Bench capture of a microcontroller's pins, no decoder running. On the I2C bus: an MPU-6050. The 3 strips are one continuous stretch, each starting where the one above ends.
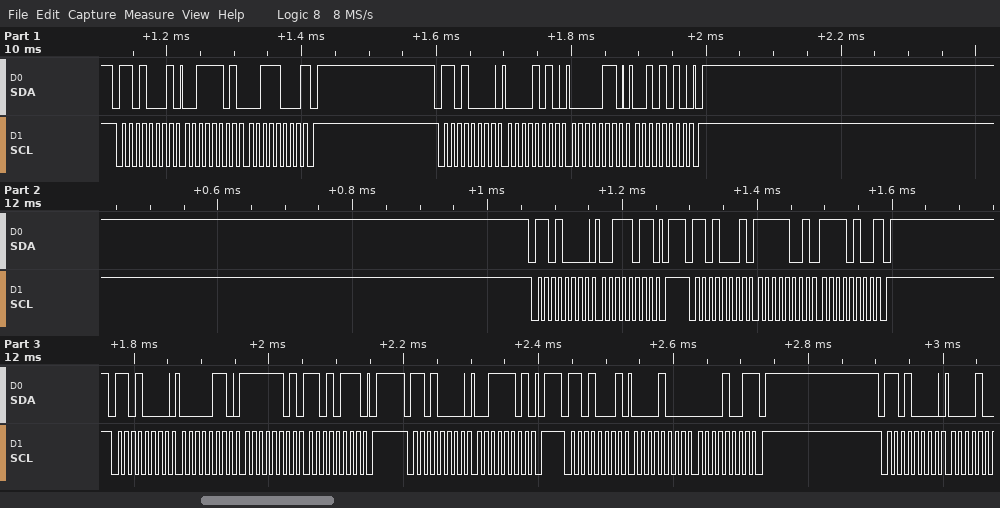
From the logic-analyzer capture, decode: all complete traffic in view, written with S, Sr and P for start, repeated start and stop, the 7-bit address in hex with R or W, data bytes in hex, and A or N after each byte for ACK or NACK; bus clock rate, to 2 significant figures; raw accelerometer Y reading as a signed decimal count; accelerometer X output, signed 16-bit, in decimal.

S 68R A 3D A 38 N P S 68W A 0A A 06 A 2A A P S 68W A 3B A P S 68R A F9 A F4 N P S 68W A 06 A FD A D7 A P S 68W A 3D A P S 68R A 08 A 09 N P S 68W A
100 kHz
2057
-1548
